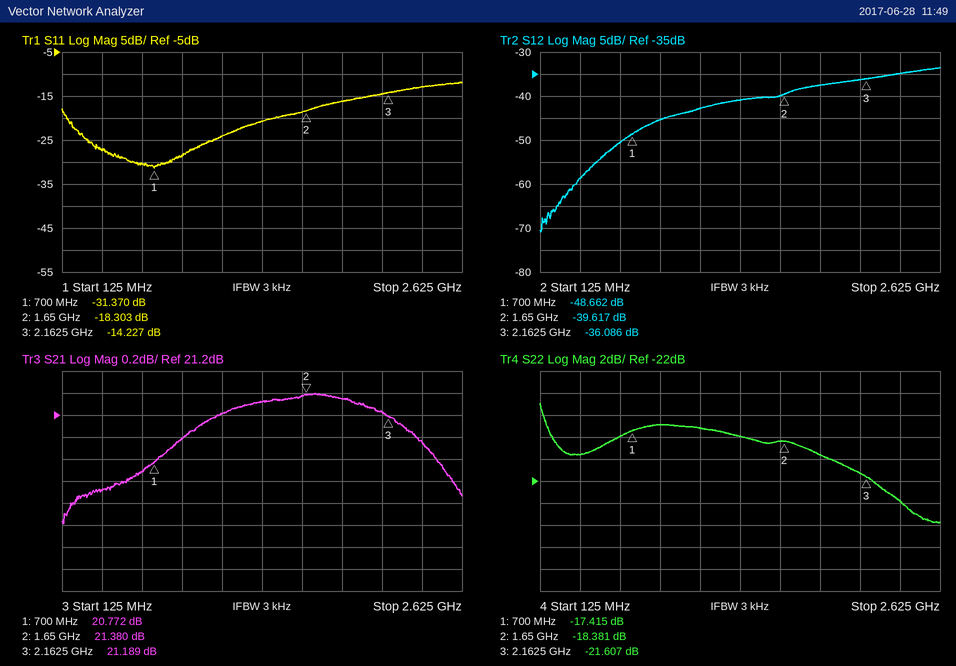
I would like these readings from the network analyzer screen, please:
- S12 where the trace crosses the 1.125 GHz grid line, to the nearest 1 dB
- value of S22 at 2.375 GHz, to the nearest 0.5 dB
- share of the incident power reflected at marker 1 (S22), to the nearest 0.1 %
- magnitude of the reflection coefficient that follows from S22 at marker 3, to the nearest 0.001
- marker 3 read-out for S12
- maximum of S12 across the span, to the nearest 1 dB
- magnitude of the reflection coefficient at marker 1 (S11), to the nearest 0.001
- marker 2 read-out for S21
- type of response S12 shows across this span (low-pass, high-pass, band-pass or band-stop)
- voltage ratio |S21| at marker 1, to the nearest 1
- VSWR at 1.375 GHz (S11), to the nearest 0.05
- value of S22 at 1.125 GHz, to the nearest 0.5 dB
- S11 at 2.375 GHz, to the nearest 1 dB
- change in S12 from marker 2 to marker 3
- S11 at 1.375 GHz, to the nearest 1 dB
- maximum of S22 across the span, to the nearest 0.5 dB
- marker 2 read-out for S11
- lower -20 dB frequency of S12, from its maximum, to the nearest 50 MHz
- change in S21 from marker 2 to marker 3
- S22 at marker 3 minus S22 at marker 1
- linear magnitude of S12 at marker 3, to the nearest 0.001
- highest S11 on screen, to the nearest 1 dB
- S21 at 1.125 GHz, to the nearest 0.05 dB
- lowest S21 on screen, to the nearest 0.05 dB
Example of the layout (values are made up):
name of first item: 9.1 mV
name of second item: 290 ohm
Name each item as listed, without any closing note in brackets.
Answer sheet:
S12 where the trace crosses the 1.125 GHz grid line, to the nearest 1 dB: -43 dB
value of S22 at 2.375 GHz, to the nearest 0.5 dB: -24.0 dB
share of the incident power reflected at marker 1 (S22), to the nearest 0.1 %: 1.8 %
magnitude of the reflection coefficient that follows from S22 at marker 3, to the nearest 0.001: 0.083
marker 3 read-out for S12: -36.086 dB
maximum of S12 across the span, to the nearest 1 dB: -34 dB
magnitude of the reflection coefficient at marker 1 (S11), to the nearest 0.001: 0.027
marker 2 read-out for S21: 21.380 dB
type of response S12 shows across this span: high-pass
voltage ratio |S21| at marker 1, to the nearest 1: 11
VSWR at 1.375 GHz (S11), to the nearest 0.05: 1.20
value of S22 at 1.125 GHz, to the nearest 0.5 dB: -17.0 dB
S11 at 2.375 GHz, to the nearest 1 dB: -13 dB
change in S12 from marker 2 to marker 3: 3.531 dB
S11 at 1.375 GHz, to the nearest 1 dB: -21 dB
maximum of S22 across the span, to the nearest 0.5 dB: -15.0 dB
marker 2 read-out for S11: -18.303 dB
lower -20 dB frequency of S12, from its maximum, to the nearest 50 MHz: 500 MHz
change in S21 from marker 2 to marker 3: -0.191 dB
S22 at marker 3 minus S22 at marker 1: -4.192 dB
linear magnitude of S12 at marker 3, to the nearest 0.001: 0.016
highest S11 on screen, to the nearest 1 dB: -12 dB
S21 at 1.125 GHz, to the nearest 0.05 dB: 21.20 dB
lowest S21 on screen, to the nearest 0.05 dB: 20.20 dB
